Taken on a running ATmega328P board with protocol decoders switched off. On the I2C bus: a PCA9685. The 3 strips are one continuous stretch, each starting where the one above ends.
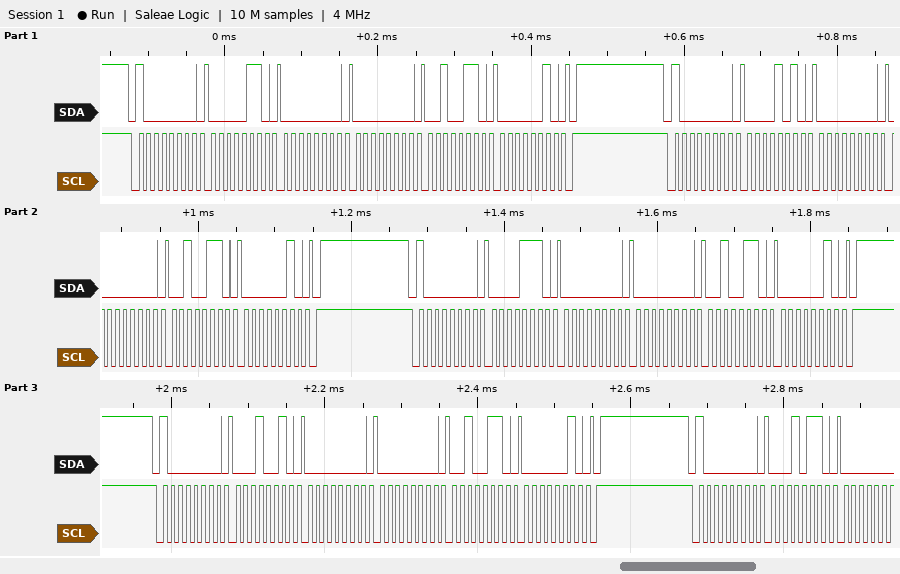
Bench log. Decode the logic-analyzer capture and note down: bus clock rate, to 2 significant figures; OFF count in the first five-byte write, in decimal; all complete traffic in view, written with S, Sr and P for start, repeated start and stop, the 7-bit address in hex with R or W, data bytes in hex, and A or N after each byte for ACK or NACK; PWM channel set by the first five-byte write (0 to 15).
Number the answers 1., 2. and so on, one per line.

1. 100 kHz
2. 550
3. S 40W A 06 A 00 A 00 A 26 A 02 A P S 40W A 0A A 00 A 00 A 26 A 02 A P S 40W A 0E A 00 A 00 A 26 A 02 A P S 40W A 12 A 00 A 00 A 26 A 02 A P S 40W A 16 A
4. 0
